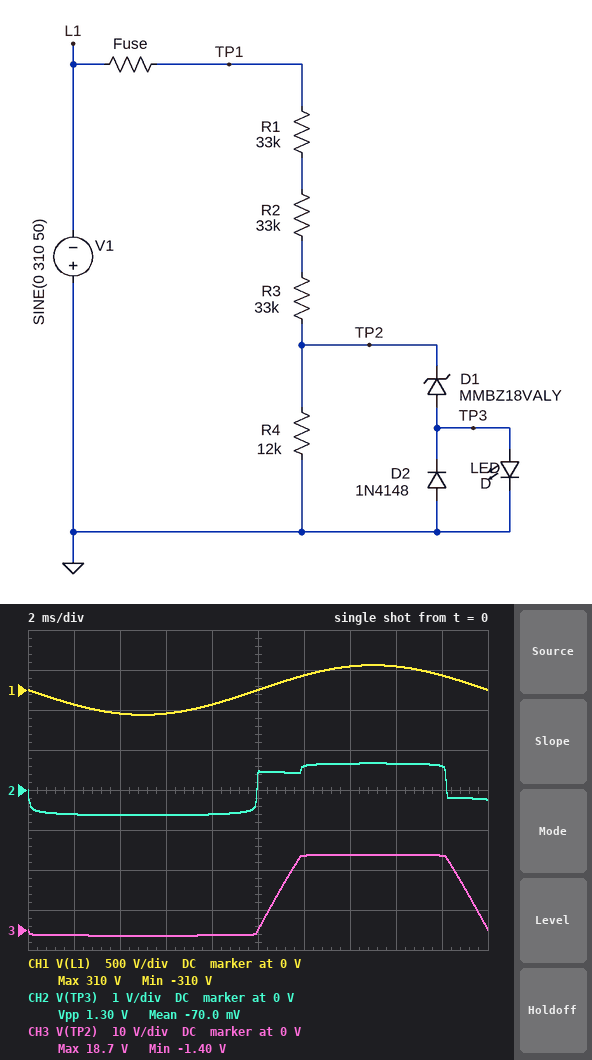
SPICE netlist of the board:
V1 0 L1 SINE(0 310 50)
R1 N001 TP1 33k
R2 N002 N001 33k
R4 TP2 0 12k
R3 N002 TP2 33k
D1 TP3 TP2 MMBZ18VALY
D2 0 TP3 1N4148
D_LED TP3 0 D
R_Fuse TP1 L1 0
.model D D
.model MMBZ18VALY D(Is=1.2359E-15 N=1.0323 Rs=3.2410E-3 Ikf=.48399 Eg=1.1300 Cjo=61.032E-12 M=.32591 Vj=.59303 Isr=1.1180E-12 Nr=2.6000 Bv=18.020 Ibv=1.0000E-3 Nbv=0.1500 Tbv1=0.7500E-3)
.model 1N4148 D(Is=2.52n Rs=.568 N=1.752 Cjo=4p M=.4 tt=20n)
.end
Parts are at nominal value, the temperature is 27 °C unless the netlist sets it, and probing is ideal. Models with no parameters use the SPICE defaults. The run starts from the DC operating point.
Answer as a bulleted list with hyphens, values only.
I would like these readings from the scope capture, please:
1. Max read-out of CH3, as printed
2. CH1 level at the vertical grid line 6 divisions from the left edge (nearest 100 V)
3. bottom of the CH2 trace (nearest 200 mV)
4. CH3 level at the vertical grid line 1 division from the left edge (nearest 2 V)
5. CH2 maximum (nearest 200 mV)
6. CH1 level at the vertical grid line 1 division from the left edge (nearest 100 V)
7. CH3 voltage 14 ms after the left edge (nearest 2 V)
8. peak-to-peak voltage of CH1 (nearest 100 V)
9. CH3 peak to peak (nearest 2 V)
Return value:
- 18.7 V
- 200 V
- -600 mV
- -2 V
- 600 mV
- -200 V
- 18 V
- 600 V
- 20 V
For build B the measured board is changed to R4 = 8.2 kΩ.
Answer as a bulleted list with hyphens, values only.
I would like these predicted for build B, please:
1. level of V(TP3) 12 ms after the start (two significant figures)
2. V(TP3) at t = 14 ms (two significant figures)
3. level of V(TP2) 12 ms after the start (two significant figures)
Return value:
- 420 mV
- 640 mV
- 14 V
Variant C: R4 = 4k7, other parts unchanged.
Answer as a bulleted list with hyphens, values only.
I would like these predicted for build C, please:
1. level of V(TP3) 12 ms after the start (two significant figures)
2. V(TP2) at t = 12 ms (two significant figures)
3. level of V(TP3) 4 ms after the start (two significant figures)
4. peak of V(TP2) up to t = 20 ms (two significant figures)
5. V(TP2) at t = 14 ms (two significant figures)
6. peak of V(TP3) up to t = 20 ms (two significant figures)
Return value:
- 410 mV
- 8.3 V
- -630 mV
- 14 V
- 13 V
- 450 mV
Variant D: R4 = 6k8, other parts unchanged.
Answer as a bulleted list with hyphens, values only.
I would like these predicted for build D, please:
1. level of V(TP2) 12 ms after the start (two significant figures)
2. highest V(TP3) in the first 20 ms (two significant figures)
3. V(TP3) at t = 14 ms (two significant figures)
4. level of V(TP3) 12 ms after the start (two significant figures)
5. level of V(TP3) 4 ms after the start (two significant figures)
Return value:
- 12 V
- 610 mV
- 580 mV
- 420 mV
- -630 mV
